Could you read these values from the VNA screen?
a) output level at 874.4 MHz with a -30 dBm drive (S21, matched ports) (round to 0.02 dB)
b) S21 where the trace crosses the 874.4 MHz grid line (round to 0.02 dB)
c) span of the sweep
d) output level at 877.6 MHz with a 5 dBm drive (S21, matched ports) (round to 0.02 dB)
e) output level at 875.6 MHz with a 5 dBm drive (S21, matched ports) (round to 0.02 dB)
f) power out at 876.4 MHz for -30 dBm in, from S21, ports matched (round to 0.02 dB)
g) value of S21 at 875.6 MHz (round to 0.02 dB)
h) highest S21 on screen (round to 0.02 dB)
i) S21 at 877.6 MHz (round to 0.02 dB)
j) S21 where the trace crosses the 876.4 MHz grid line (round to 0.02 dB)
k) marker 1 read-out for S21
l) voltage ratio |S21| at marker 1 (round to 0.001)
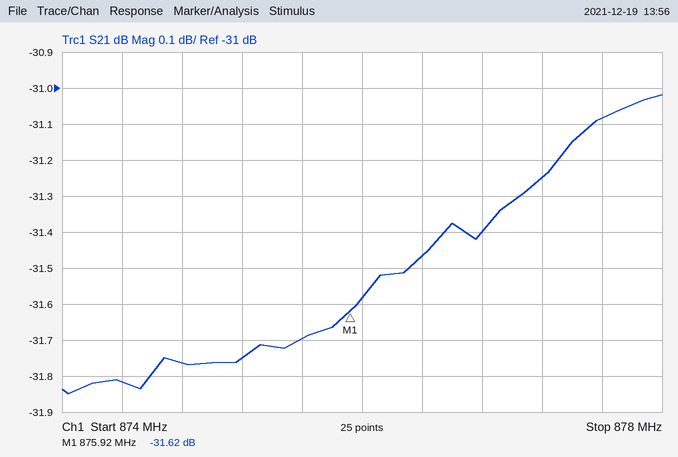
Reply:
-61.82 dBm
-31.82 dB
4 MHz
-26.08 dBm
-26.70 dBm
-61.46 dBm
-31.70 dB
-31.02 dB
-31.08 dB
-31.46 dB
-31.62 dB
0.026
